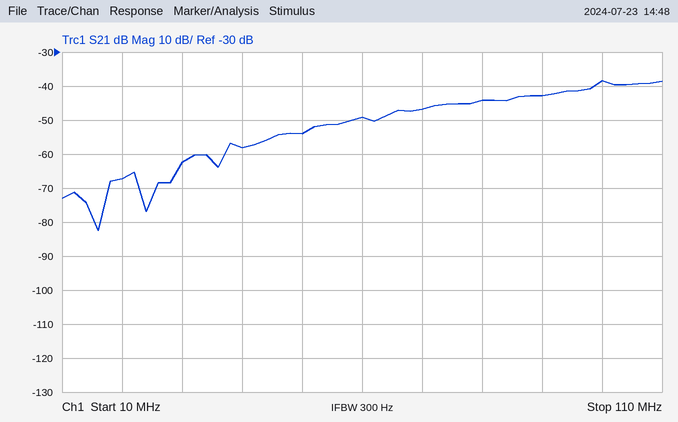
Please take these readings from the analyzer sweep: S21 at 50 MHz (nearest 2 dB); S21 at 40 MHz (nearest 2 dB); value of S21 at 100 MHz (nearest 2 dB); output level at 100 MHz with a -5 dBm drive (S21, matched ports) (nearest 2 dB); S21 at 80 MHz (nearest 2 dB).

-54 dB
-58 dB
-38 dB
-44 dBm
-44 dB
